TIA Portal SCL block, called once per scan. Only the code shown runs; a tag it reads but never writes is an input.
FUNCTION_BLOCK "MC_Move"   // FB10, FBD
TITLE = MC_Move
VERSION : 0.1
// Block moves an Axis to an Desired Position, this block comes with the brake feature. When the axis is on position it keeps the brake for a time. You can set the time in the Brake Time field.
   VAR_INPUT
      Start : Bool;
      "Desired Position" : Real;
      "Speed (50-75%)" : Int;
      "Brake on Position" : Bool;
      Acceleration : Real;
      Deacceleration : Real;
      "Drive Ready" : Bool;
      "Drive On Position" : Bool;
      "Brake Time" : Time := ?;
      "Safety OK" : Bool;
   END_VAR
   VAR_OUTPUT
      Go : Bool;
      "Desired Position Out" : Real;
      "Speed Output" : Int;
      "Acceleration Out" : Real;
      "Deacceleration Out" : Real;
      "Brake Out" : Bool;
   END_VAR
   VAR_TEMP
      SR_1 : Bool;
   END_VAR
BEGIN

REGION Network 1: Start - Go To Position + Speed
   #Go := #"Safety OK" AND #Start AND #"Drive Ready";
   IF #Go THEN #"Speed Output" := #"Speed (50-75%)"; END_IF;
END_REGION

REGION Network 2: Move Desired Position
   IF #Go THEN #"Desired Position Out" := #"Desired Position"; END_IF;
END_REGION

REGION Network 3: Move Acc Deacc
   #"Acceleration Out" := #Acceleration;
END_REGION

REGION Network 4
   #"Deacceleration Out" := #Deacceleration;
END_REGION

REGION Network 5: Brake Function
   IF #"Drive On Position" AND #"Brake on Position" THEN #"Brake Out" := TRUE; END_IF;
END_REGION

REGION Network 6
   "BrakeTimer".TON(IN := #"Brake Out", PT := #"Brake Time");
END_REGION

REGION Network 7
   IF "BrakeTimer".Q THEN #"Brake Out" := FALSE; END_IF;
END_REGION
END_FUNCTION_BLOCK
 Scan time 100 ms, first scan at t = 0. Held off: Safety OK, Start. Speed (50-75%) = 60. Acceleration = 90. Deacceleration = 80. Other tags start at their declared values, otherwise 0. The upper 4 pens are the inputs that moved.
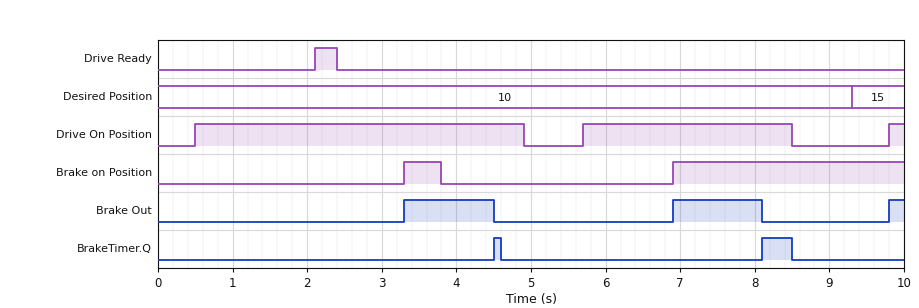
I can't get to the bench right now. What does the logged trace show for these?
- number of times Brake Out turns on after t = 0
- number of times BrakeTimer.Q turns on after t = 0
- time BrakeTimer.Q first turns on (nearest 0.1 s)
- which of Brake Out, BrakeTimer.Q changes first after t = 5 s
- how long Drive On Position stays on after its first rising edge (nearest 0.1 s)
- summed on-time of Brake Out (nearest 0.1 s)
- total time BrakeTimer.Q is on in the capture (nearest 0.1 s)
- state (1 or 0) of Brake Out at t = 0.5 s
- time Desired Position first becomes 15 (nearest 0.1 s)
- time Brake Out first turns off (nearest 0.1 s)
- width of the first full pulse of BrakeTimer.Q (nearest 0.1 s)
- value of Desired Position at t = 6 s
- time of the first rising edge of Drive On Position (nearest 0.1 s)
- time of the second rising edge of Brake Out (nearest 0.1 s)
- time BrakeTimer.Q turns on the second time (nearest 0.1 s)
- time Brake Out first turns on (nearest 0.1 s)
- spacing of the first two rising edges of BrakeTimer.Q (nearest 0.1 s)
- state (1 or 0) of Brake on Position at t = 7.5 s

3
2
4.5 s
Brake Out
4.4 s
2.6 s
0.5 s
0
9.3 s
4.5 s
0.1 s
10
0.5 s
6.9 s
8.1 s
3.3 s
3.6 s
1
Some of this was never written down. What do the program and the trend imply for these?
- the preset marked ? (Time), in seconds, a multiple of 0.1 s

1.2 s
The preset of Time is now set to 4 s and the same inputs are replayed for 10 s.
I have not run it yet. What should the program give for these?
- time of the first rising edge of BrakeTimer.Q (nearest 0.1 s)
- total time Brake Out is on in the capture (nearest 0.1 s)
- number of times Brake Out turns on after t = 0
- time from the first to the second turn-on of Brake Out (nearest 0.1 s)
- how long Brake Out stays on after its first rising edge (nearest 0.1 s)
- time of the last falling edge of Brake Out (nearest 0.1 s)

7.3 s
4.2 s
2
6.5 s
4.0 s
7.3 s
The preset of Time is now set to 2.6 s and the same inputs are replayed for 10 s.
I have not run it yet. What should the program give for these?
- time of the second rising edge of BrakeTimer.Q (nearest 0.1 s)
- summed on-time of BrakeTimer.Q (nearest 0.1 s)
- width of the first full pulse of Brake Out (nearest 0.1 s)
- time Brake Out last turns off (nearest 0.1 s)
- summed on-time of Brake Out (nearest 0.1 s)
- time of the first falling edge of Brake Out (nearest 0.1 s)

9.5 s
0.2 s
2.6 s
9.5 s
5.4 s
5.9 s
